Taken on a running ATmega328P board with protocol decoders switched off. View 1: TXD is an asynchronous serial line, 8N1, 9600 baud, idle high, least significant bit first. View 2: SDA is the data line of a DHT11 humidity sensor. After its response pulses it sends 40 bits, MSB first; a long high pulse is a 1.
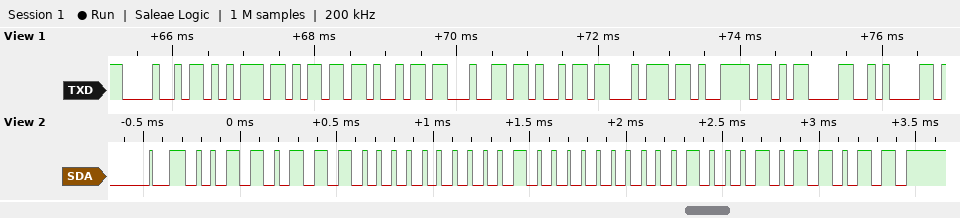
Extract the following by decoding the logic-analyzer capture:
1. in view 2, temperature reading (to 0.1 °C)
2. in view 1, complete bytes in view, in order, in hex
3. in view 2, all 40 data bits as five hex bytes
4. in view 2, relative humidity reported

32.4 °C
48 75 6D 69 64 69 74 79 0D 0A
37 00 20 04 5B
55 %
